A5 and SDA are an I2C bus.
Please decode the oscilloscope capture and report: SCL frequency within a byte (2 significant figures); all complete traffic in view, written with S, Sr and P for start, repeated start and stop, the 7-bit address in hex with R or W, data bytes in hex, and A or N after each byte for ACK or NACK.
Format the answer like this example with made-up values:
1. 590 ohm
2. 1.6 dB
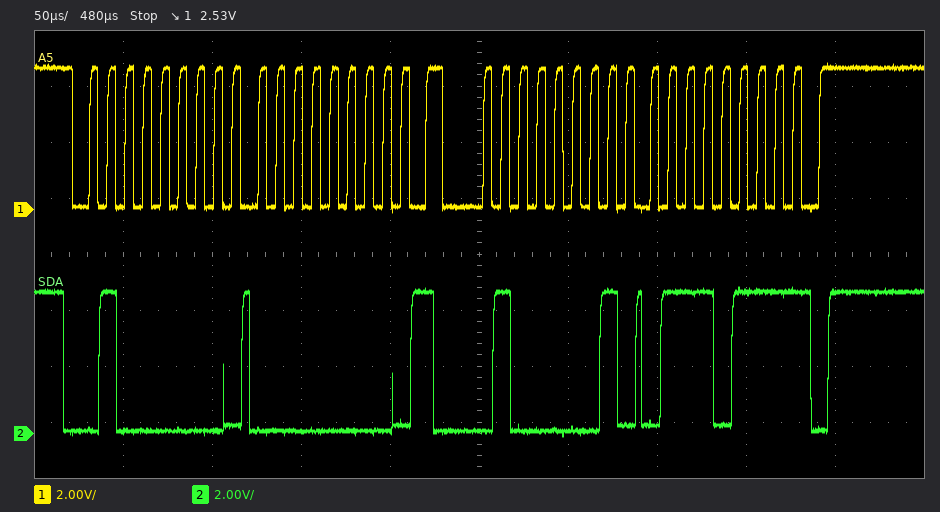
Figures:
1. 100 kHz
2. S 20W A 00 A Sr 20R A 77 N P
